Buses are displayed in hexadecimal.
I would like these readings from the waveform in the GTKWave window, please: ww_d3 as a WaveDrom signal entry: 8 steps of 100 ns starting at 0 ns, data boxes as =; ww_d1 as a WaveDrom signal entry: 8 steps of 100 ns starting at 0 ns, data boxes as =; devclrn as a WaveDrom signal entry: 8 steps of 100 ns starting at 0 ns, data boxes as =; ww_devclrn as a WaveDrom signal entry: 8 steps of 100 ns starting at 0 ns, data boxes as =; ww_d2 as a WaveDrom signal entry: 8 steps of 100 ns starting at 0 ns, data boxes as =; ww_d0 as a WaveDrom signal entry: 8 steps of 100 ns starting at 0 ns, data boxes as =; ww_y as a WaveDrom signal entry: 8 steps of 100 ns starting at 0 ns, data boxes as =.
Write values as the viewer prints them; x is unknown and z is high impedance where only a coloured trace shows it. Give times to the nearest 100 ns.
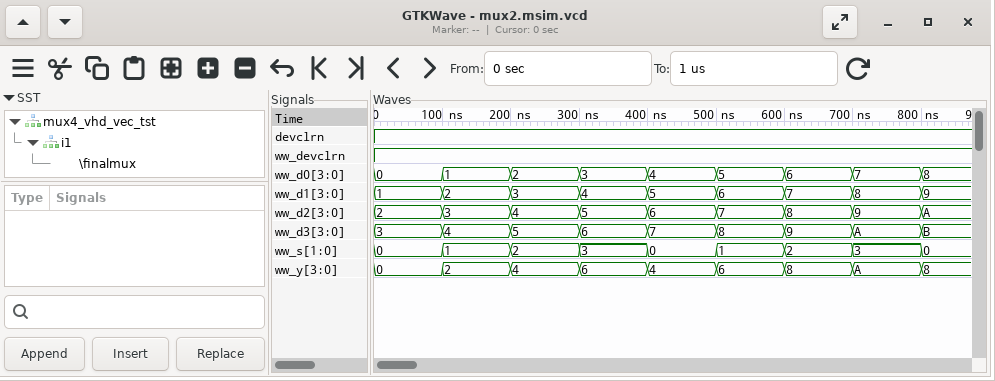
{name: 'ww_d3', wave: '========', data: '3 4 5 6 7 8 9 A'}
{name: 'ww_d1', wave: '========', data: '1 2 3 4 5 6 7 8'}
{name: 'devclrn', wave: '1.......'}
{name: 'ww_devclrn', wave: '1.......'}
{name: 'ww_d2', wave: '========', data: '2 3 4 5 6 7 8 9'}
{name: 'ww_d0', wave: '========', data: '0 1 2 3 4 5 6 7'}
{name: 'ww_y', wave: '========', data: '0 2 4 6 4 6 8 A'}
